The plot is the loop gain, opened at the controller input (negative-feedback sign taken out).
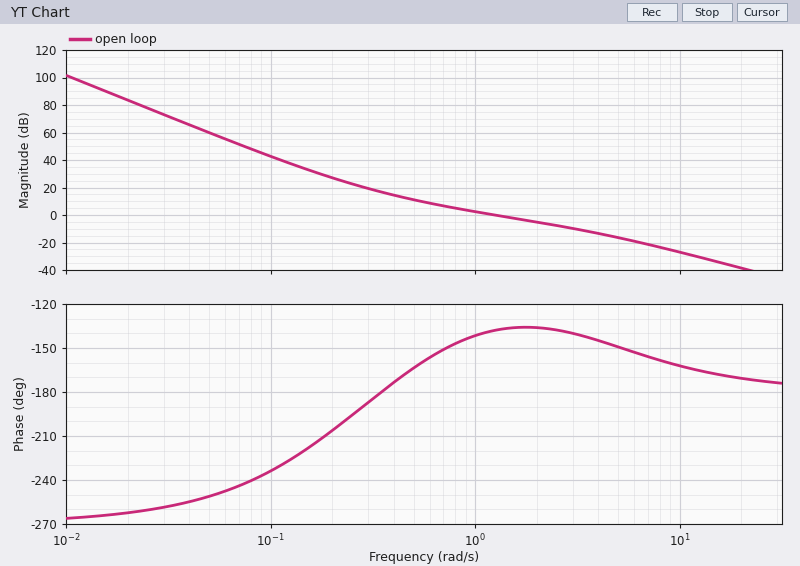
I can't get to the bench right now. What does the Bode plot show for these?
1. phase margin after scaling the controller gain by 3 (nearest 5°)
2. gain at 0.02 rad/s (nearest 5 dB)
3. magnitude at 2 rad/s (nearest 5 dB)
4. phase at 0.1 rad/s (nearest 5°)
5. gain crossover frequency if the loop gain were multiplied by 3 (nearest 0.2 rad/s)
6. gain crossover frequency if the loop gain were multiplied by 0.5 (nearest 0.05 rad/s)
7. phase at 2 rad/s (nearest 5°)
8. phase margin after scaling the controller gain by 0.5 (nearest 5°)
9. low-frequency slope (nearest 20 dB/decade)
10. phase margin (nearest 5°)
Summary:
40°
85 dB
-5 dB
-235°
3.0 rad/s
0.75 rad/s
-135°
30°
-60 dB/decade
40°
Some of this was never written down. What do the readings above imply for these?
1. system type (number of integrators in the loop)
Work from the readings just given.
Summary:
3
